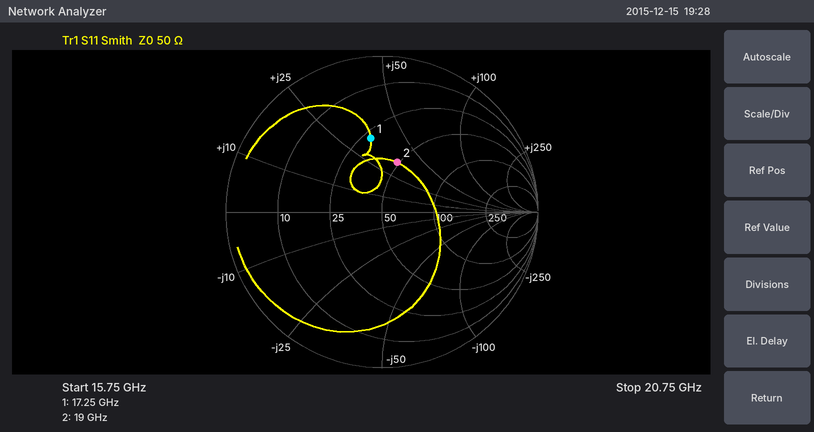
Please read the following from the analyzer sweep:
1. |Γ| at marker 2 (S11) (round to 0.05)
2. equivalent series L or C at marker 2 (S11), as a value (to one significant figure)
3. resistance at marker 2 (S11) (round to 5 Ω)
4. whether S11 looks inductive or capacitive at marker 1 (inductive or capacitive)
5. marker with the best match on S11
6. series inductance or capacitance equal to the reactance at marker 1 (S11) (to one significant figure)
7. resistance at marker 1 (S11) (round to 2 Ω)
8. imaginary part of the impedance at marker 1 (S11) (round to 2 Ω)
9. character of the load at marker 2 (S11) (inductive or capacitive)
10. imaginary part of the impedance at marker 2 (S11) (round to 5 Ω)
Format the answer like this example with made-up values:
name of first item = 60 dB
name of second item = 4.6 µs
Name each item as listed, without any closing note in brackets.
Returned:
|Γ| at marker 2 (S11) = 0.35
equivalent series L or C at marker 2 (S11), as a value = 300 pH
resistance at marker 2 (S11) = 50 Ω
whether S11 looks inductive or capacitive at marker 1 = inductive
marker with the best match on S11 = marker 2
series inductance or capacitance equal to the reactance at marker 1 (S11) = 300 pH
resistance at marker 1 (S11) = 28 Ω
imaginary part of the impedance at marker 1 (S11) = +34 Ω
character of the load at marker 2 (S11) = inductive
imaginary part of the impedance at marker 2 (S11) = +35 Ω
